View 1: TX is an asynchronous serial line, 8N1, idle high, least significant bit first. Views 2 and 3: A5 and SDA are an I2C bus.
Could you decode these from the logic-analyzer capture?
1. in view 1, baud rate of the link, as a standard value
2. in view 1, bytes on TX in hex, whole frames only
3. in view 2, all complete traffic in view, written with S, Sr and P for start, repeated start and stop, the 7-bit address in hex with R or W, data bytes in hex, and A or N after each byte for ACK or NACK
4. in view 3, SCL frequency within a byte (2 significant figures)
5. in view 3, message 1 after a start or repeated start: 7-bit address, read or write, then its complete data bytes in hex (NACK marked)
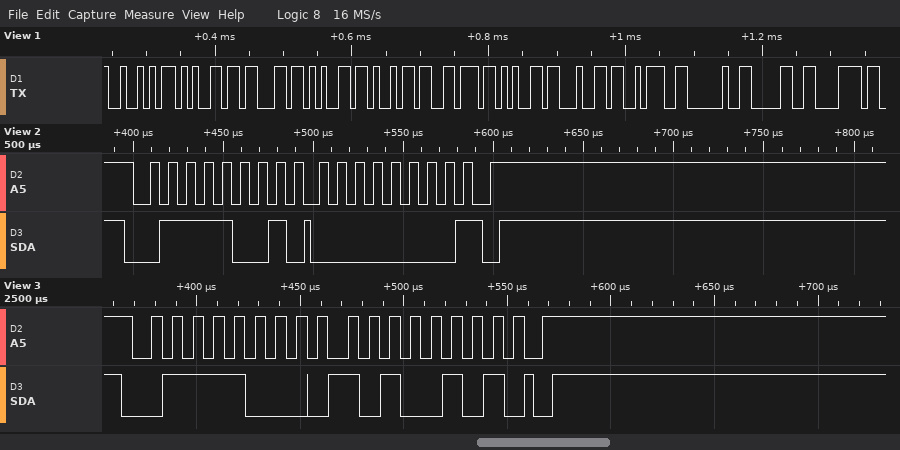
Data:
115200 baud
52 65 63 65 69 76 65 64 3A 20 30 78
S 3CR A 00 N P
100 kHz
0x3C write: A5
